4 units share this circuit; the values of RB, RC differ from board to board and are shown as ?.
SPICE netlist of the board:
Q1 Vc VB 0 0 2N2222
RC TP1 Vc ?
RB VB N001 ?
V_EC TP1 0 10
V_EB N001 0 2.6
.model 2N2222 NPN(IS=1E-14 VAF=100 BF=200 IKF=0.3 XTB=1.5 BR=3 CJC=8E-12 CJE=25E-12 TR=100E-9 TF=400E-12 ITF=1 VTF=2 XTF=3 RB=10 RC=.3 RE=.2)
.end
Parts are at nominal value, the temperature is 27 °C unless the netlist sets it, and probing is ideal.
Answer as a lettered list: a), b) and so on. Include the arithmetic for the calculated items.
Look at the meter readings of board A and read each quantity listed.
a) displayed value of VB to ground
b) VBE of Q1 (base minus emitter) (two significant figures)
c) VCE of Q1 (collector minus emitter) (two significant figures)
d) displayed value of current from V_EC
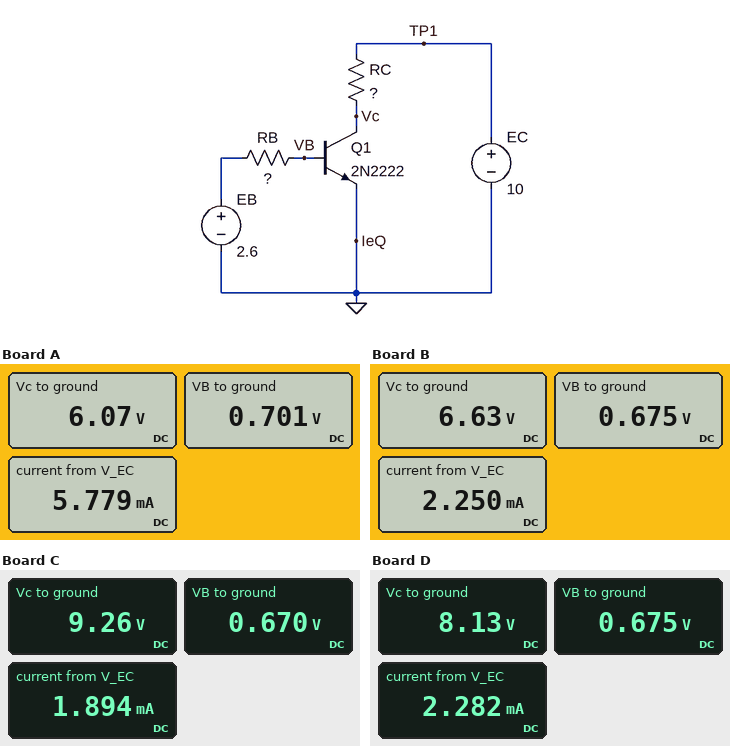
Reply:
a) 0.701 V
b) 701 mV = 700 mV
c) 6.07 V = 6.1 V
d) 5.779 mA
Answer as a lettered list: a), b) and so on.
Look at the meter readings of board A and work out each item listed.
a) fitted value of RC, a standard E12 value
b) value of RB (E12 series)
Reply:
a) 680 Ω
b) 68 kΩ
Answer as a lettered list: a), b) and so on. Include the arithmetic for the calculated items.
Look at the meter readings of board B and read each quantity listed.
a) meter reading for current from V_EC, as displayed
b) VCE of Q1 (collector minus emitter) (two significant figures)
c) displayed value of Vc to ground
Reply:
a) 2.250 mA
b) 6.63 V = 6.6 V
c) 6.63 V
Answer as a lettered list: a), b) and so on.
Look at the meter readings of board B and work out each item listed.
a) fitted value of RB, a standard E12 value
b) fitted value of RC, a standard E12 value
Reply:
a) 180 kΩ
b) 1.5 kΩ
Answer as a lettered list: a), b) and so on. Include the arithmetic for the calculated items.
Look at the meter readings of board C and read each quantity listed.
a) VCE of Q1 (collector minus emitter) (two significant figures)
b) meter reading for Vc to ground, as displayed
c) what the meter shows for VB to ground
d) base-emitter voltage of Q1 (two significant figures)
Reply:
a) 9.26 V = 9.3 V
b) 9.26 V
c) 0.670 V
d) 670 mV = 670 mV
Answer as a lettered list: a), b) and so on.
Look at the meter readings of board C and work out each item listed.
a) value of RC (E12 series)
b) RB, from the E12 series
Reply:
a) 390 Ω
b) 220 kΩ
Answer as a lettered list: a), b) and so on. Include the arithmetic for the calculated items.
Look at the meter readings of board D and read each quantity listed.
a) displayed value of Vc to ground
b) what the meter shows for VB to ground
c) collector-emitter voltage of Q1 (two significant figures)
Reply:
a) 8.13 V
b) 0.675 V
c) 8.13 V = 8.1 V
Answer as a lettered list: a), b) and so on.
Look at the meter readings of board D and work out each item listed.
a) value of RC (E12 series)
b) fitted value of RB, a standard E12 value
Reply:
a) 820 Ω
b) 180 kΩ
